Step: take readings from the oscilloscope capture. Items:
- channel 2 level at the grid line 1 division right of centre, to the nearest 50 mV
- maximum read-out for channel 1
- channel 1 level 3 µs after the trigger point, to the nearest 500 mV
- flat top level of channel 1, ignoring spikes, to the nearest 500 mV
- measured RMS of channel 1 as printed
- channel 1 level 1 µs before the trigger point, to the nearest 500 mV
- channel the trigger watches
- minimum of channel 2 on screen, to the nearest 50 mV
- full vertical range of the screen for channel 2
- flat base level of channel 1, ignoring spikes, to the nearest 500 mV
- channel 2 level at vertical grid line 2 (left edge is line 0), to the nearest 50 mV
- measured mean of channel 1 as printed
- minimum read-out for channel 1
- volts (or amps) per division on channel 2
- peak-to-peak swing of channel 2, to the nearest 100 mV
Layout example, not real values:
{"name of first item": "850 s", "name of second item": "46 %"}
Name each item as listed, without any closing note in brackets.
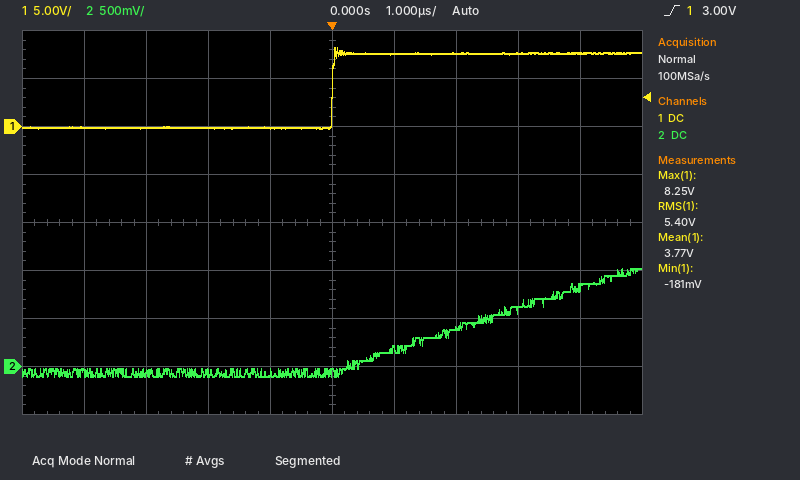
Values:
{"channel 2 level at the grid line 1 division right of centre, to the nearest 50 mV": "200 mV", "maximum read-out for channel 1": "8.25 V", "channel 1 level 3 µs after the trigger point, to the nearest 500 mV": "7.5 V", "flat top level of channel 1, ignoring spikes, to the nearest 500 mV": "7.5 V", "measured RMS of channel 1 as printed": "5.40 V", "channel 1 level 1 µs before the trigger point, to the nearest 500 mV": "0.0 V", "channel the trigger watches": "channel 1", "minimum of channel 2 on screen, to the nearest 50 mV": "-100 mV", "full vertical range of the screen for channel 2": "4 V", "flat base level of channel 1, ignoring spikes, to the nearest 500 mV": "0.0 V", "channel 2 level at vertical grid line 2 (left edge is line 0), to the nearest 50 mV": "-50 mV", "measured mean of channel 1 as printed": "3.77 V", "minimum read-out for channel 1": "-181 mV", "volts (or amps) per division on channel 2": "500 mV", "peak-to-peak swing of channel 2, to the nearest 100 mV": "1.10 V"}
